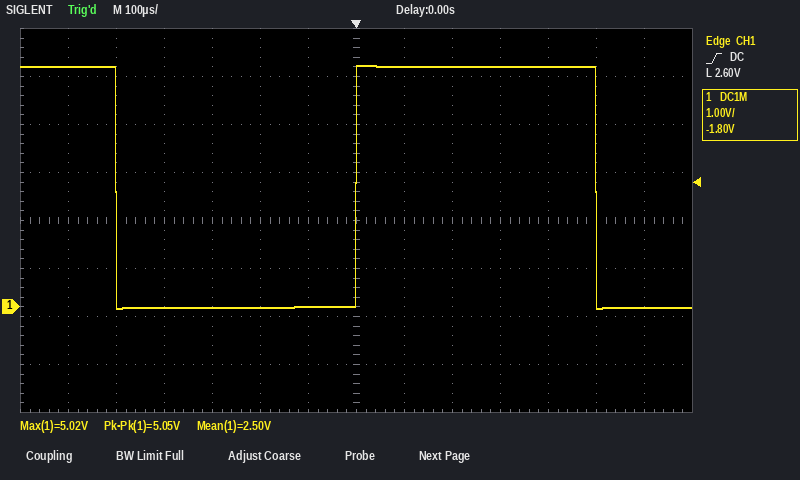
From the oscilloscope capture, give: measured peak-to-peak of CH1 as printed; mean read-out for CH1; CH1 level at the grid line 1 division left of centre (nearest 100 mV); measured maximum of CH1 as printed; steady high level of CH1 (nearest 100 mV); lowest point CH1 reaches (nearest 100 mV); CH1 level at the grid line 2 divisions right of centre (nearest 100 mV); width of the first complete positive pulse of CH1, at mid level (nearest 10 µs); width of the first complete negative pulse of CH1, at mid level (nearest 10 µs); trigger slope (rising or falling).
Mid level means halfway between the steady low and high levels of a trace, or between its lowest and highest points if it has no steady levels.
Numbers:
5.05 V
2.50 V
0.0 V
5.02 V
5.0 V
0.0 V
5.0 V
500 µs
500 µs
rising
